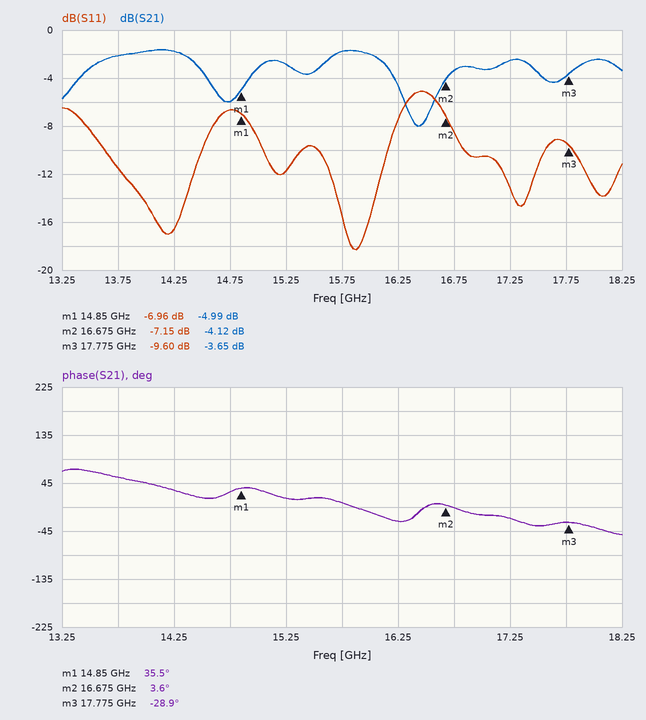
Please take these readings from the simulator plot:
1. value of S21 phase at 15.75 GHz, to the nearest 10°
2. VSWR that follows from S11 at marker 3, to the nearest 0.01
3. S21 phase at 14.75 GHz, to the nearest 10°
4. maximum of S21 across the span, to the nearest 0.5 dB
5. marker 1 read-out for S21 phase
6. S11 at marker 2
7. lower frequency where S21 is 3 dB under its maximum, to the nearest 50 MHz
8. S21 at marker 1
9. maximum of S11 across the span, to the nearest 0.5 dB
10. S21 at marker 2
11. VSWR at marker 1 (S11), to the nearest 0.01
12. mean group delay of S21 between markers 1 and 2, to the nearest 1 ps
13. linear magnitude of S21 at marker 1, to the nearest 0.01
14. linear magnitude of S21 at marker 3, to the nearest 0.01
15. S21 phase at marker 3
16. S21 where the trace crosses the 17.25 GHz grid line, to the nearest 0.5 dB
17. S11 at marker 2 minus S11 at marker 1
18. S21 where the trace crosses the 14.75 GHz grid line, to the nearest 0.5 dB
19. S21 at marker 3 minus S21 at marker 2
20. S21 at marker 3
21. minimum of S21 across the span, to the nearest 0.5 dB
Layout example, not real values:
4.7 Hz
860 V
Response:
10°
1.99
30°
-1.5 dB
35.5°
-7.15 dB
13.35 GHz
-4.99 dB
-5.0 dB
-4.12 dB
2.63
49 ps
0.56
0.66
-28.9°
-2.5 dB
-0.19 dB
-6.0 dB
0.47 dB
-3.65 dB
-8.0 dB
